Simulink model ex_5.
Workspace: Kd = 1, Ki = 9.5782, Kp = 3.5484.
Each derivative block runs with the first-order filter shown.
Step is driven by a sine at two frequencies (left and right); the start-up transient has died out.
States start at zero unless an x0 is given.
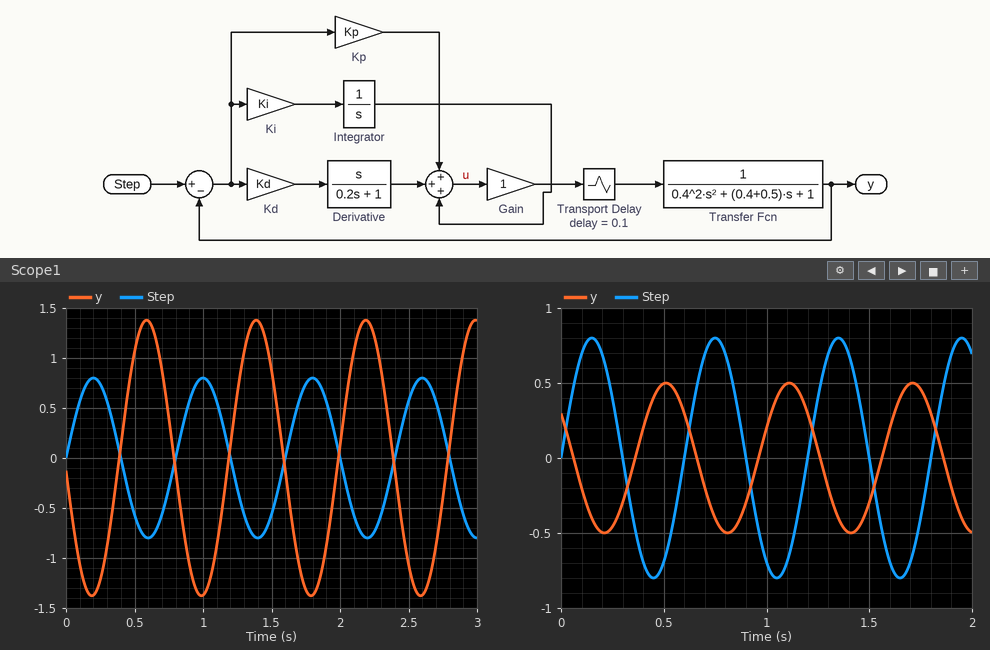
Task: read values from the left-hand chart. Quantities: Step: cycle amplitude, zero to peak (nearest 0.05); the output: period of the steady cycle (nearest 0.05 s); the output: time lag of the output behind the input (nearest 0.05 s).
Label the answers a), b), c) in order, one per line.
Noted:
a) 0.80
b) 0.80 s
c) 0.40 s
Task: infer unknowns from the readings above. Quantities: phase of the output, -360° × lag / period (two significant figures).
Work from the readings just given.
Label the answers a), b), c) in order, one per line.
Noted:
a) -180°
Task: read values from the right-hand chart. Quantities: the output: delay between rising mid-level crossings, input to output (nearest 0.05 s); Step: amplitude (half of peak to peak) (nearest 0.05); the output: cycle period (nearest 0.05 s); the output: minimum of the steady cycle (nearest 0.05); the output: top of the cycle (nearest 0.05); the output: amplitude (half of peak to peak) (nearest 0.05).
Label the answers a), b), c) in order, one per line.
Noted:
a) 0.35 s
b) 0.80
c) 0.60 s
d) -0.50
e) 0.50
f) 0.50
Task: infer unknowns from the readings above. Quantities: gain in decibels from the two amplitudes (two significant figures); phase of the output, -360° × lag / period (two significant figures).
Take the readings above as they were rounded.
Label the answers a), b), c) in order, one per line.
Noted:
a) -4.1 dB
b) -210°
